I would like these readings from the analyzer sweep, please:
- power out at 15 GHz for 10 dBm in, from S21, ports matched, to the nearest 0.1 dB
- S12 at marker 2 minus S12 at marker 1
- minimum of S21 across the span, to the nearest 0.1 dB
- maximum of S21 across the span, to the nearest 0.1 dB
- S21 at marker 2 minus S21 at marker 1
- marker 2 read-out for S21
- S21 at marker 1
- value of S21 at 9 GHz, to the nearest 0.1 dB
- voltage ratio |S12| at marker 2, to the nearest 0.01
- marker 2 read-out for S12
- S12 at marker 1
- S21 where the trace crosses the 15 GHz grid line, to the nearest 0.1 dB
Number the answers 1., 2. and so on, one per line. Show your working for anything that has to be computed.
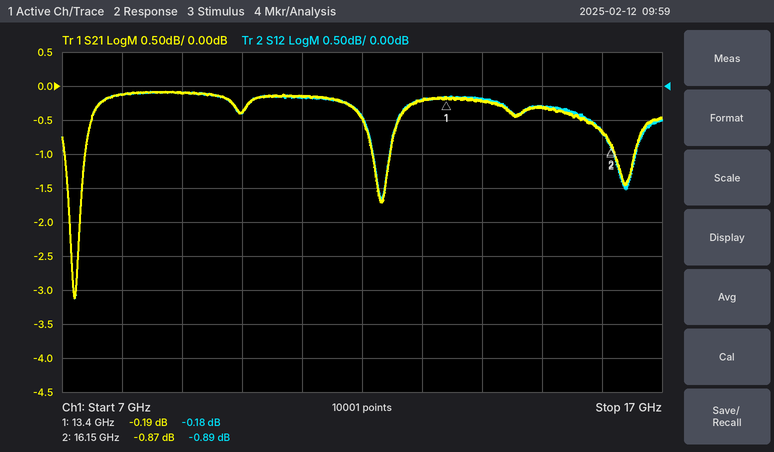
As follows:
1. 10 dBm + (-0.3 dB) = 9.7 dBm
2. -0.89 − (-0.18) = -0.71 dB
3. -3.1 dB
4. -0.1 dB
5. -0.87 − (-0.19) = -0.68 dB
6. -0.87 dB
7. -0.19 dB
8. -0.1 dB
9. 10^(-0.89/20) ≈ 0.90
10. -0.89 dB
11. -0.18 dB
12. -0.3 dB
